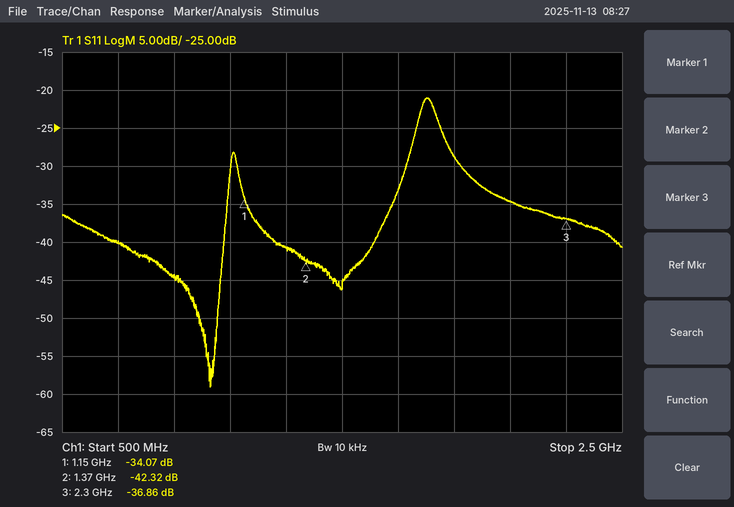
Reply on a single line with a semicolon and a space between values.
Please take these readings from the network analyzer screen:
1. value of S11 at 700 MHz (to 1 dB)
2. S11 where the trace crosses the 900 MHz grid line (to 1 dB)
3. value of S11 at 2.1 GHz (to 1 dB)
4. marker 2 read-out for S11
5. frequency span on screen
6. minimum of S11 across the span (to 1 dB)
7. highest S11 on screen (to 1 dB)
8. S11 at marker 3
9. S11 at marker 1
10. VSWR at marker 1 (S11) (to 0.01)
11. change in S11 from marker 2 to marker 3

-40 dB; -45 dB; -35 dB; -42.32 dB; 2 GHz; -59 dB; -21 dB; -36.86 dB; -34.07 dB; 1.04; 5.46 dB
